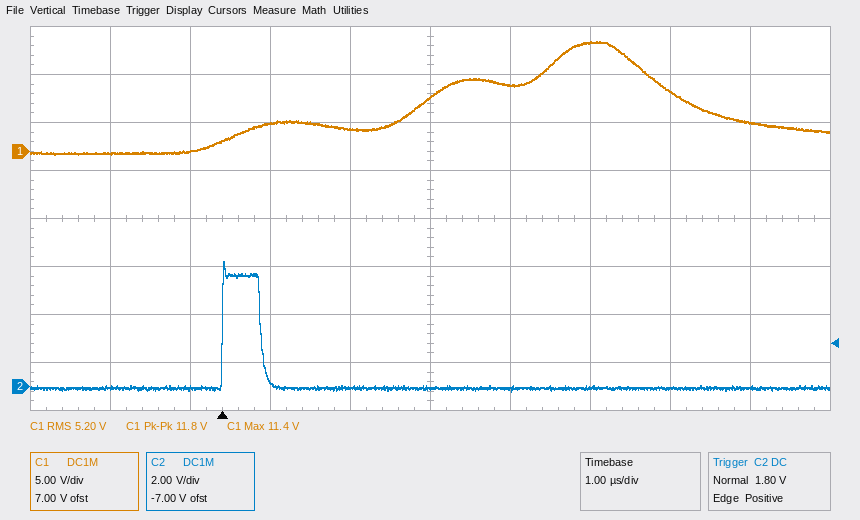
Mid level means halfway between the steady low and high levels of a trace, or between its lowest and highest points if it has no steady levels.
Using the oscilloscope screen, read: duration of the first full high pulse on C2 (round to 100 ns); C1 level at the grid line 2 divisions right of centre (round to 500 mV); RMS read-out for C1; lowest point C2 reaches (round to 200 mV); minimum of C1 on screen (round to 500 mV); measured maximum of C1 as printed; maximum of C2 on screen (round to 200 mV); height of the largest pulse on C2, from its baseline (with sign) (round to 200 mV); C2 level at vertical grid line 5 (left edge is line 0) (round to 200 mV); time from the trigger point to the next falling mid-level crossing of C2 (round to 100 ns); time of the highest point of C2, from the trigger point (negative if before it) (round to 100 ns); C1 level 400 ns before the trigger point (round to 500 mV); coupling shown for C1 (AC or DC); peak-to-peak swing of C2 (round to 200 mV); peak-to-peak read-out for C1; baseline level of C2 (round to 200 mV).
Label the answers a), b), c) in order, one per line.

a) 500 ns
b) 11.5 V
c) 5.20 V
d) -200 mV
e) -500 mV
f) 11.4 V
g) 5.2 V
h) +5.2 V
i) 0.0 V
j) 500 ns
k) 0.0 µs
l) 0.0 V
m) DC
n) 5.4 V
o) 11.8 V
p) 0.0 V
